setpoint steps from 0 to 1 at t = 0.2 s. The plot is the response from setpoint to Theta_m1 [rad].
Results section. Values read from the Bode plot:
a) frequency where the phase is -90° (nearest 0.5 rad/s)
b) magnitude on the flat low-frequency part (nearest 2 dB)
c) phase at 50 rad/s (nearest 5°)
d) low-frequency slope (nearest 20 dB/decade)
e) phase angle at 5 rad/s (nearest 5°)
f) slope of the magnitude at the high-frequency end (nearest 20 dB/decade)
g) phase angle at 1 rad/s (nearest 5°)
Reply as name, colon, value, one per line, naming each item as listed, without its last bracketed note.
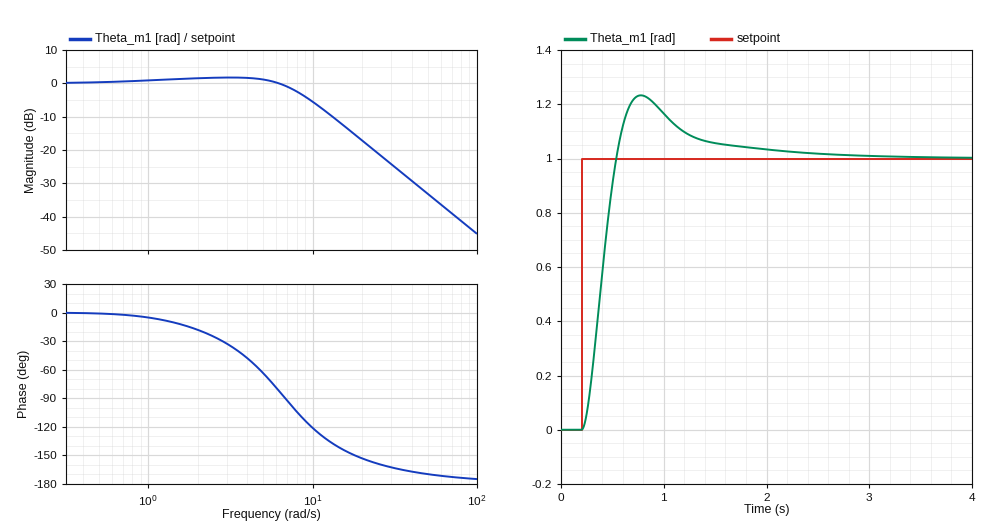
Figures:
frequency where the phase is -90°: 7.0 rad/s
magnitude on the flat low-frequency part: 0 dB
phase at 50 rad/s: -170°
low-frequency slope: 0 dB/decade
phase angle at 5 rad/s: -65°
slope of the magnitude at the high-frequency end: -40 dB/decade
phase angle at 1 rad/s: -5°
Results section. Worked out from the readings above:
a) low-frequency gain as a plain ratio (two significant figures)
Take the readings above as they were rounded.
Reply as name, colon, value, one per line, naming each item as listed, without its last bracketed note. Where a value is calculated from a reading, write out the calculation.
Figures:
low-frequency gain as a plain ratio: 10^(0 / 20) = 1.0
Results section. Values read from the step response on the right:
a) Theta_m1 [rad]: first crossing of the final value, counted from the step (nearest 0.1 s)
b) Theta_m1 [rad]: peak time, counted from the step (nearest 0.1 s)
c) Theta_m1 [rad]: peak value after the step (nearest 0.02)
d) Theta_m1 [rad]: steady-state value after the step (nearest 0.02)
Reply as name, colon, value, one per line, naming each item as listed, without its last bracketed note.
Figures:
Theta_m1 [rad]: first crossing of the final value, counted from the step: 0.3 s
Theta_m1 [rad]: peak time, counted from the step: 0.6 s
Theta_m1 [rad]: peak value after the step: 1.24
Theta_m1 [rad]: steady-state value after the step: 1.00
